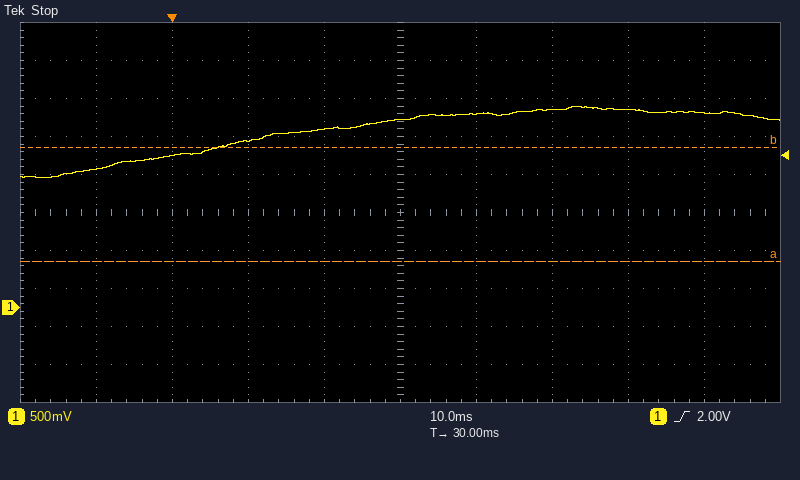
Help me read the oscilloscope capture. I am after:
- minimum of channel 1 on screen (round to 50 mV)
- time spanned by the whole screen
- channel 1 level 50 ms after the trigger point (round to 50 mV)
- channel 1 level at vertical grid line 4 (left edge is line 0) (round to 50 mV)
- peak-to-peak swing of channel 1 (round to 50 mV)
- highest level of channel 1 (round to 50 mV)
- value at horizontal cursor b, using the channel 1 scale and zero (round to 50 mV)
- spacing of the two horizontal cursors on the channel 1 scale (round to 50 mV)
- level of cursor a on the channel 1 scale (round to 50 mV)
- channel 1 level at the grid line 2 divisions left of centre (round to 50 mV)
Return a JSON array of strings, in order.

["1.70 V", "100 ms", "2.60 V", "2.35 V", "950 mV", "2.65 V", "2.10 V", "1.50 V", "600 mV", "2.20 V"]
